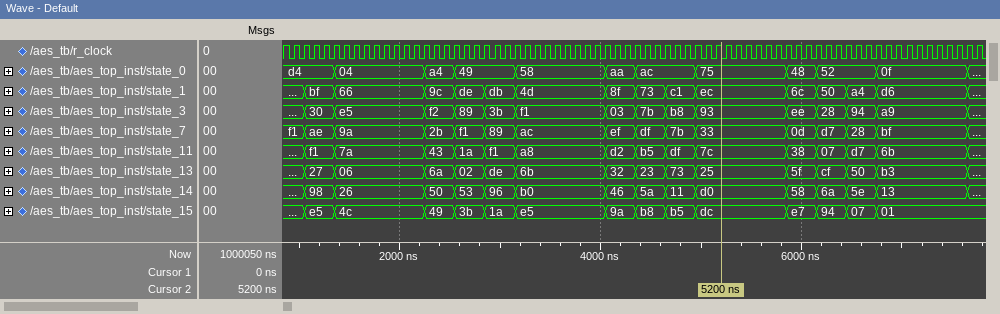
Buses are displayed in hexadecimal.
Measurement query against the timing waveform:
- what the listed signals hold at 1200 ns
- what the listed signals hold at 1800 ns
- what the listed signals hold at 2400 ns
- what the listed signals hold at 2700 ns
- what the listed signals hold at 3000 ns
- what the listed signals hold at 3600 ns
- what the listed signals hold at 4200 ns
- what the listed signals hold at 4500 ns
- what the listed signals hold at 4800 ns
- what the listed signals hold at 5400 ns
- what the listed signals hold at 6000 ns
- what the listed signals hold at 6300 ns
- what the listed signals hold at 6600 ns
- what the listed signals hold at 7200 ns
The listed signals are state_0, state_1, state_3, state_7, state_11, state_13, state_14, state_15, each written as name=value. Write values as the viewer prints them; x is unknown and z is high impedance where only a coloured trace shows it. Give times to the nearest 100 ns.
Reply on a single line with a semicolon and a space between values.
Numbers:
state_0=d4, state_1=bf, state_3=30, state_7=ae, state_11=f1, state_13=27, state_14=98, state_15=e5; state_0=04, state_1=66, state_3=e5, state_7=9a, state_11=7a, state_13=06, state_14=26, state_15=4c; state_0=a4, state_1=9c, state_3=f2, state_7=2b, state_11=43, state_13=6a, state_14=50, state_15=49; state_0=49, state_1=de, state_3=89, state_7=f1, state_11=1a, state_13=02, state_14=53, state_15=3b; state_0=49, state_1=db, state_3=3b, state_7=89, state_11=f1, state_13=de, state_14=96, state_15=1a; state_0=58, state_1=4d, state_3=f1, state_7=ac, state_11=a8, state_13=6b, state_14=b0, state_15=e5; state_0=aa, state_1=8f, state_3=03, state_7=ef, state_11=d2, state_13=32, state_14=46, state_15=9a; state_0=ac, state_1=73, state_3=7b, state_7=df, state_11=b5, state_13=23, state_14=5a, state_15=b8; state_0=ac, state_1=c1, state_3=b8, state_7=7b, state_11=df, state_13=73, state_14=11, state_15=b5; state_0=75, state_1=ec, state_3=93, state_7=33, state_11=7c, state_13=25, state_14=d0, state_15=dc; state_0=48, state_1=6c, state_3=ee, state_7=0d, state_11=38, state_13=5f, state_14=58, state_15=e7; state_0=52, state_1=50, state_3=28, state_7=d7, state_11=07, state_13=cf, state_14=6a, state_15=94; state_0=52, state_1=a4, state_3=94, state_7=28, state_11=d7, state_13=50, state_14=5e, state_15=07; state_0=0f, state_1=d6, state_3=a9, state_7=bf, state_11=6b, state_13=b3, state_14=13, state_15=01
